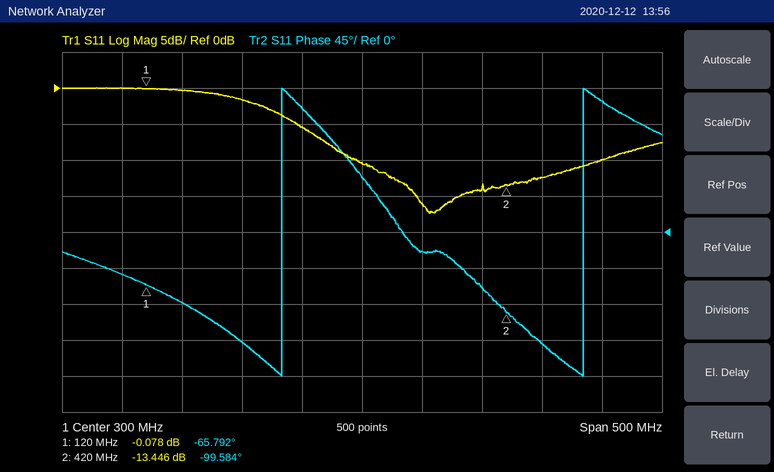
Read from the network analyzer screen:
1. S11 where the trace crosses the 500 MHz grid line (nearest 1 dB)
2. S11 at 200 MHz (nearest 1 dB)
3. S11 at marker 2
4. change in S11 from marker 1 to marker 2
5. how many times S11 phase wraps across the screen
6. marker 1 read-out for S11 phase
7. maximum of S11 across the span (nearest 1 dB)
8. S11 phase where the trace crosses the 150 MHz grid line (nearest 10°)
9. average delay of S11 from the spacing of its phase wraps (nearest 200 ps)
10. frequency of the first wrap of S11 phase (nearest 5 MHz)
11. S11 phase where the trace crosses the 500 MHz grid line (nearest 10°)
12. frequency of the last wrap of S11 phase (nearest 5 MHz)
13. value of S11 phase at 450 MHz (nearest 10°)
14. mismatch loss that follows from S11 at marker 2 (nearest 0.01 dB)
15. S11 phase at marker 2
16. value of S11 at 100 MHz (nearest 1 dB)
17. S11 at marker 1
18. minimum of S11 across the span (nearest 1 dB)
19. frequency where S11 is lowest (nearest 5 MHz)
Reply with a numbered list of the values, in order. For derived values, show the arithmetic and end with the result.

1. -10 dB
2. -2 dB
3. -13.446 dB
4. -13.446 − (-0.078) = -13.368 dB
5. 2
6. -65.792°
7. 0 dB
8. -90°
9. 1 cycle / (485 MHz − 235 MHz) ≈ 4.0 ns
10. 235 MHz
11. 160°
12. 485 MHz
13. -140°
14. −10 log10(1 − 10^(-13.446/10)) ≈ 0.20 dB
15. -99.584°
16. 0 dB
17. -0.078 dB
18. -17 dB
19. 355 MHz
